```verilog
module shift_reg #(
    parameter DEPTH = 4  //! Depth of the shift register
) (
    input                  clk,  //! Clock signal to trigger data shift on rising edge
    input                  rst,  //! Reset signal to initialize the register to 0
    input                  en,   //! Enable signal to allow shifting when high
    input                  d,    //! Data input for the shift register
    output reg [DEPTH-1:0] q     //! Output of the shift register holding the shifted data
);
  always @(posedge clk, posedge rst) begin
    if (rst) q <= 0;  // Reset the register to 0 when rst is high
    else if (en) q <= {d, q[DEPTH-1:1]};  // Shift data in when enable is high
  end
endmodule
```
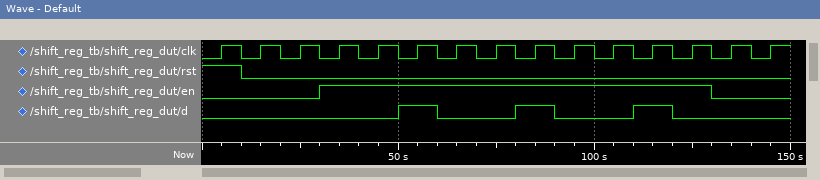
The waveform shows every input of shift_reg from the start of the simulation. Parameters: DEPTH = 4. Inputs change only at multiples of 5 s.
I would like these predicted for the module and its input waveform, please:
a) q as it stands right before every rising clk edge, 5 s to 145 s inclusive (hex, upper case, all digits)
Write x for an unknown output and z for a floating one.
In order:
0, 0, 0, 0, 0, 0, 8, 4, 2, 9, 4, 2, 9, 4, 4
